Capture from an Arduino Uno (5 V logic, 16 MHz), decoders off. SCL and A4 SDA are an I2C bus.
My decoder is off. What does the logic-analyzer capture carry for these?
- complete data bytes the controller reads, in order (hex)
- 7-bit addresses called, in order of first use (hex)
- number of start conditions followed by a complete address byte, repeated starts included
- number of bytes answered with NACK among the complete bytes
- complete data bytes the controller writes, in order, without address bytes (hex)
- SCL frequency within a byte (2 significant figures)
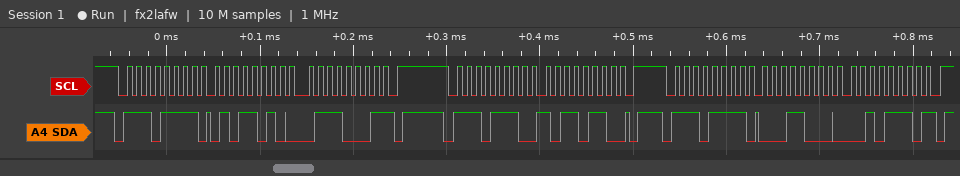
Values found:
5A 71 18 2E
0x77
3
2
B6
100 kHz
